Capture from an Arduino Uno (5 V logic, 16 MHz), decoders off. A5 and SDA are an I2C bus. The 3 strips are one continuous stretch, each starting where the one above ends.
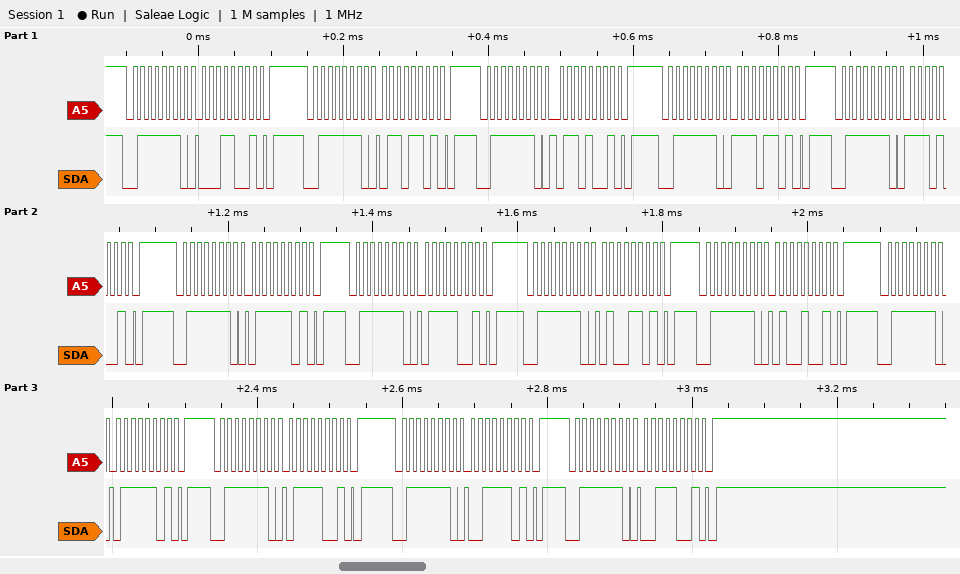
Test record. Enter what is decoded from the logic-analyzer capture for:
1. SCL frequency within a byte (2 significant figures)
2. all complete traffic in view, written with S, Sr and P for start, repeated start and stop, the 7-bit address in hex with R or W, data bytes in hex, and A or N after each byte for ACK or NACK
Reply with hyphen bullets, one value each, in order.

- 100 kHz
- S 3FW A 19 A P S 3FW A 6D A P S 3FW A 69 A P S 3FW A ED A P S 3FW A E9 A P S 3FW A 7D A P S 3FW A 79 A P S 3FW A 4D A P S 3FW A 49 A P S 3FW A 7D A P S 3FW A 79 A P S 3FW A 3D A P S 3FW A 39 A P
